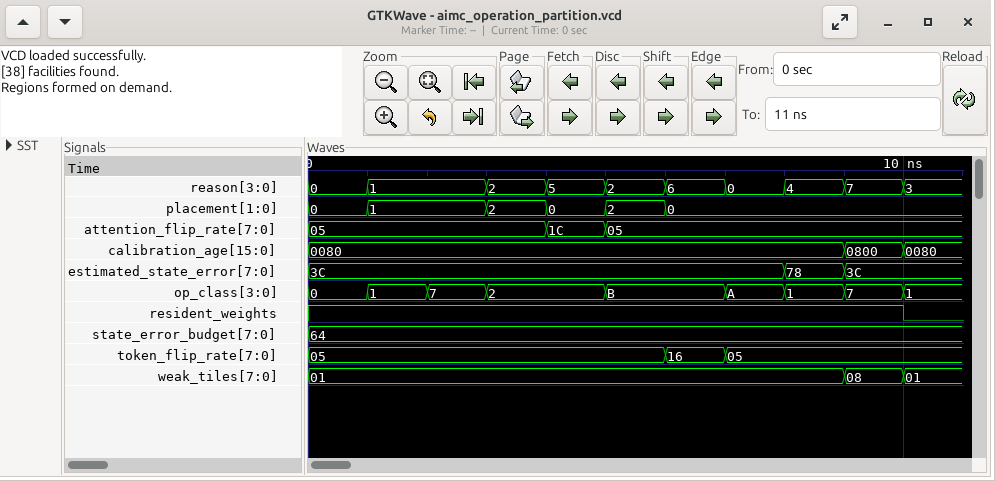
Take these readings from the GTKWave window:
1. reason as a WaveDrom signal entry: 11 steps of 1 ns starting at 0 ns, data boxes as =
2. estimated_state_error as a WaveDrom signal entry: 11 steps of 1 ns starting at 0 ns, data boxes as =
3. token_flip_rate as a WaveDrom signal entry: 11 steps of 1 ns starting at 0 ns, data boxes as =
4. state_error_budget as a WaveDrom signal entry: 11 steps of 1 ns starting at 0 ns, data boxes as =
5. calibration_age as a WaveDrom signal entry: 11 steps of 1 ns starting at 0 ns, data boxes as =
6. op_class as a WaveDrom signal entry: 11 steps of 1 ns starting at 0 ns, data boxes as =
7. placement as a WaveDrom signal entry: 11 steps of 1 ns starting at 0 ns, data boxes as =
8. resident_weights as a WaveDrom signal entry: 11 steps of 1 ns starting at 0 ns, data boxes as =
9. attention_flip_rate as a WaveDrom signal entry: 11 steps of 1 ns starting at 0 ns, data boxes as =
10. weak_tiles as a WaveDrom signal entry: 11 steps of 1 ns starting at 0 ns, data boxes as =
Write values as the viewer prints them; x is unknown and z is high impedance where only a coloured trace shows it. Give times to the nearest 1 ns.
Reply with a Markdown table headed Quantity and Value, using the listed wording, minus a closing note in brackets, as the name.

| Quantity | Value |
|---|---|
| reason as a WaveDrom signal entry: 11 steps of 1 ns starting at 0 ns, data boxes as = | {name: 'reason', wave: '==.========', data: '0 1 2 5 2 6 0 4 7 3'} |
| estimated_state_error as a WaveDrom signal entry: 11 steps of 1 ns starting at 0 ns, data boxes as = | {name: 'estimated_state_error', wave: '=.......==.', data: '3C 78 3C'} |
| token_flip_rate as a WaveDrom signal entry: 11 steps of 1 ns starting at 0 ns, data boxes as = | {name: 'token_flip_rate', wave: '=.....==...', data: '05 16 05'} |
| state_error_budget as a WaveDrom signal entry: 11 steps of 1 ns starting at 0 ns, data boxes as = | {name: 'state_error_budget', wave: '=..........', data: '64'} |
| calibration_age as a WaveDrom signal entry: 11 steps of 1 ns starting at 0 ns, data boxes as = | {name: 'calibration_age', wave: '=........==', data: '0080 0800 0080'} |
| op_class as a WaveDrom signal entry: 11 steps of 1 ns starting at 0 ns, data boxes as = | {name: 'op_class', wave: '====.=.====', data: '0 1 7 2 B A 1 7 1'} |
| placement as a WaveDrom signal entry: 11 steps of 1 ns starting at 0 ns, data boxes as = | {name: 'placement', wave: '==.====....', data: '0 1 2 0 2 0'} |
| resident_weights as a WaveDrom signal entry: 11 steps of 1 ns starting at 0 ns, data boxes as = | {name: 'resident_weights', wave: '1.........0'} |
| attention_flip_rate as a WaveDrom signal entry: 11 steps of 1 ns starting at 0 ns, data boxes as = | {name: 'attention_flip_rate', wave: '=...==.....', data: '05 1C 05'} |
| weak_tiles as a WaveDrom signal entry: 11 steps of 1 ns starting at 0 ns, data boxes as = | {name: 'weak_tiles', wave: '=........==', data: '01 08 01'} |
